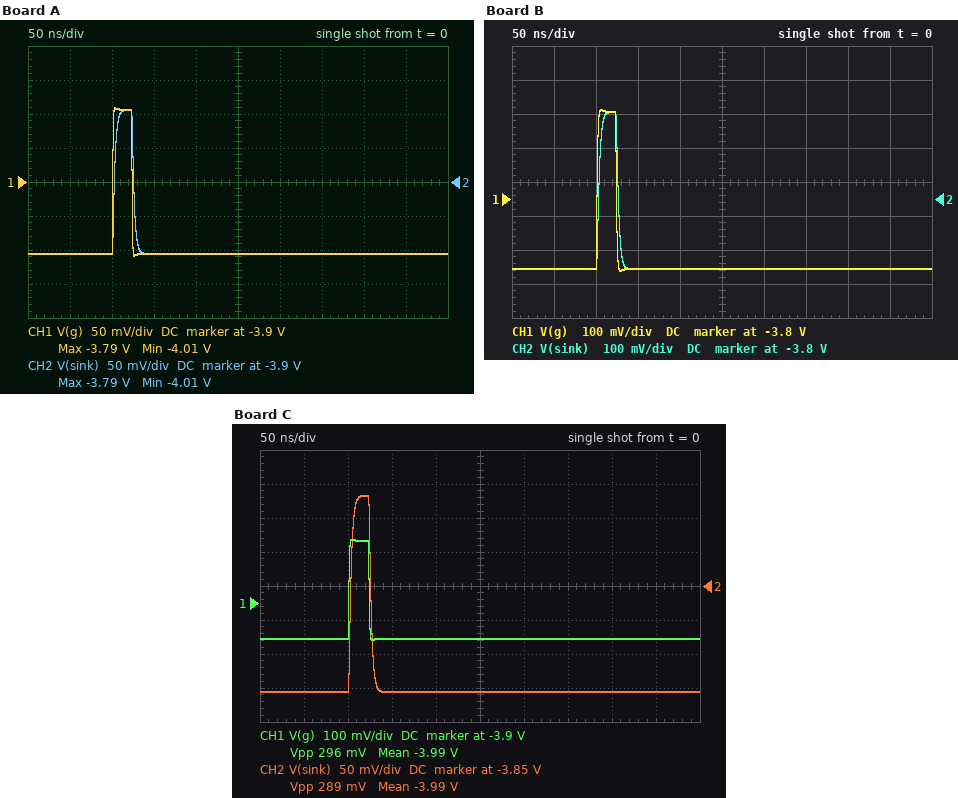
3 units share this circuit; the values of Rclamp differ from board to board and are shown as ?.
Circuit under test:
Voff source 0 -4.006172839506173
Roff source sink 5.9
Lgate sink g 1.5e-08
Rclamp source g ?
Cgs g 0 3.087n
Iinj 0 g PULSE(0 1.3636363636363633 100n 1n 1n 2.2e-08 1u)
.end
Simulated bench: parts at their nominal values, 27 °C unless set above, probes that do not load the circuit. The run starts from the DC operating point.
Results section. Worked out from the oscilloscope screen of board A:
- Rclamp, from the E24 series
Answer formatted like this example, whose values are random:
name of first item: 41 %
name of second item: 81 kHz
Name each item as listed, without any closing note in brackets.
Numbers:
Rclamp, from the E24 series: 0.16 Ω
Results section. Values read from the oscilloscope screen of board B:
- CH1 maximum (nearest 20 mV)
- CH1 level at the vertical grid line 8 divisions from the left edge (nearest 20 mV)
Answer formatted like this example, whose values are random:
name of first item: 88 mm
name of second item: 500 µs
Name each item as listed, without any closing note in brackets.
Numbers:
CH1 maximum: -3.54 V
CH1 level at the vertical grid line 8 divisions from the left edge: -4.00 V
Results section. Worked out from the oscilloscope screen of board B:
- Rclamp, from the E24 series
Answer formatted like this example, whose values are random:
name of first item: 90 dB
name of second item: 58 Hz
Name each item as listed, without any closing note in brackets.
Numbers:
Rclamp, from the E24 series: 0.36 Ω
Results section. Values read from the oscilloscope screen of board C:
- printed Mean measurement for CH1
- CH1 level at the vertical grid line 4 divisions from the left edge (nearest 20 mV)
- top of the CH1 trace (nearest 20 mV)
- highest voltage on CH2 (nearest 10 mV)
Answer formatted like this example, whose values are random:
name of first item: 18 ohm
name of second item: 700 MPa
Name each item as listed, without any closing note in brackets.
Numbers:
printed Mean measurement for CH1: -3.99 V
CH1 level at the vertical grid line 4 divisions from the left edge: -4.00 V
top of the CH1 trace: -3.72 V
highest voltage on CH2: -3.72 V
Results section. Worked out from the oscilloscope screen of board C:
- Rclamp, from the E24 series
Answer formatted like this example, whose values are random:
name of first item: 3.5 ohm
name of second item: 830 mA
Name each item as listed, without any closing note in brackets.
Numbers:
Rclamp, from the E24 series: 0.22 Ω
